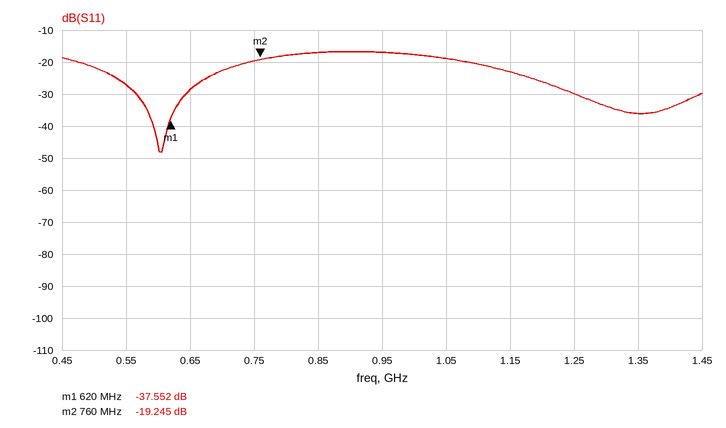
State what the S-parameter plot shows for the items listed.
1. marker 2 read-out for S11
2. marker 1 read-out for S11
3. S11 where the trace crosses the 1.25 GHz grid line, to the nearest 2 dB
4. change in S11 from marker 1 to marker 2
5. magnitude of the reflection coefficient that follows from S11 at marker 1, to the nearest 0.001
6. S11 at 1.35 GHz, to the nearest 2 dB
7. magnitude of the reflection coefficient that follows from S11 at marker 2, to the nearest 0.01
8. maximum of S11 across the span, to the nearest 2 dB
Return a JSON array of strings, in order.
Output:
["-19.245 dB", "-37.552 dB", "-30 dB", "18.307 dB", "0.013", "-36 dB", "0.11", "-16 dB"]
